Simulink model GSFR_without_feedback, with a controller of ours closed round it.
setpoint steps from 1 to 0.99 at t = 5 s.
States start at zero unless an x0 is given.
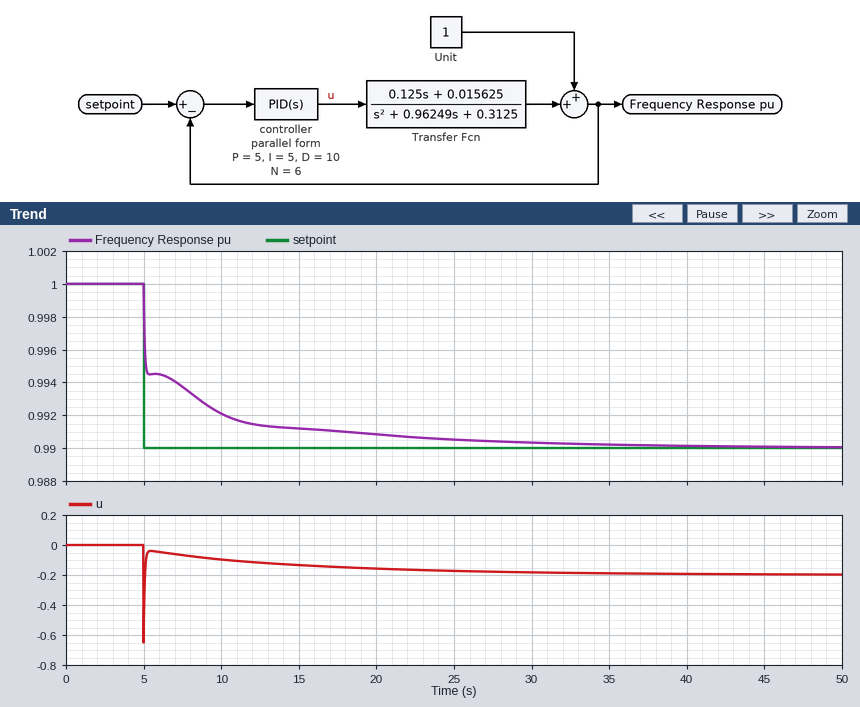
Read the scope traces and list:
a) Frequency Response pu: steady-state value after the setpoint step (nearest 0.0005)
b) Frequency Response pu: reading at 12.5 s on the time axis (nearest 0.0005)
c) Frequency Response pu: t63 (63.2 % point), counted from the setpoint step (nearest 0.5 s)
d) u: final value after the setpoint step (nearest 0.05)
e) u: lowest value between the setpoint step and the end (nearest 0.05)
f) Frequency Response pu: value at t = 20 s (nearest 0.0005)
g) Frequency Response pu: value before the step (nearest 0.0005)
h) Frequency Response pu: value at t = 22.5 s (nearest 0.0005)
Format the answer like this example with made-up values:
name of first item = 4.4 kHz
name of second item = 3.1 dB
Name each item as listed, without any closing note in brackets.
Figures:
Frequency Response pu: steady-state value after the setpoint step = 0.9900
Frequency Response pu: reading at 12.5 s on the time axis = 0.9915
Frequency Response pu: t63 (63.2 % point), counted from the setpoint step = 2.5 s
u: final value after the setpoint step = -0.20
u: lowest value between the setpoint step and the end = -0.65
Frequency Response pu: value at t = 20 s = 0.9910
Frequency Response pu: value before the step = 1.0000
Frequency Response pu: value at t = 22.5 s = 0.9905
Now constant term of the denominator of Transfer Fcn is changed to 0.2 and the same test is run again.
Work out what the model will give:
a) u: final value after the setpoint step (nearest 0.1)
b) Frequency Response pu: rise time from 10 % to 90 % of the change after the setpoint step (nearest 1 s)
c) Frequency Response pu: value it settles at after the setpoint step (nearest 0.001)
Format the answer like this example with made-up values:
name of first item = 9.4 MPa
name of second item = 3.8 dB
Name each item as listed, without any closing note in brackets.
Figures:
u: final value after the setpoint step = -0.1
Frequency Response pu: rise time from 10 % to 90 % of the change after the setpoint step = 6 s
Frequency Response pu: value it settles at after the setpoint step = 0.990
